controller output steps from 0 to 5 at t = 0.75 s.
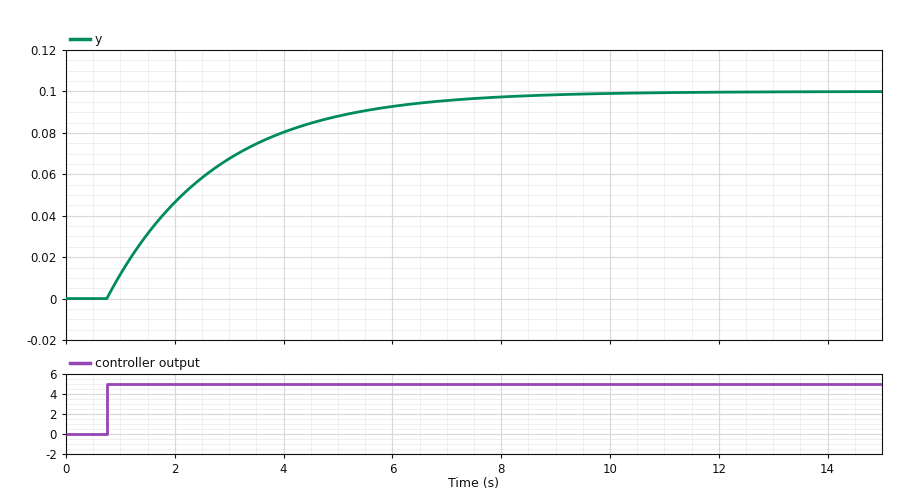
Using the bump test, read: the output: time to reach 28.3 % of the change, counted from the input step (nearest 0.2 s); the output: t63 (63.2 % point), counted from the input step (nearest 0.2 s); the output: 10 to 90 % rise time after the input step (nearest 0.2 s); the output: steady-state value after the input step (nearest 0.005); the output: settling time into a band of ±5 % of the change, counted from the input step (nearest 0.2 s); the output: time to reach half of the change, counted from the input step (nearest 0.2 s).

0.6 s
2.0 s
4.4 s
0.100
6.0 s
1.4 s
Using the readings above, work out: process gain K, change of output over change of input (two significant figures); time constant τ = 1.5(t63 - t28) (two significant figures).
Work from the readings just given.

0.020
2.1 s
